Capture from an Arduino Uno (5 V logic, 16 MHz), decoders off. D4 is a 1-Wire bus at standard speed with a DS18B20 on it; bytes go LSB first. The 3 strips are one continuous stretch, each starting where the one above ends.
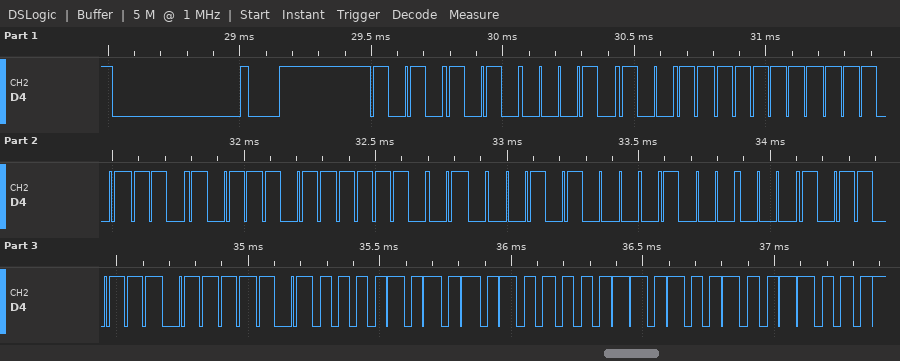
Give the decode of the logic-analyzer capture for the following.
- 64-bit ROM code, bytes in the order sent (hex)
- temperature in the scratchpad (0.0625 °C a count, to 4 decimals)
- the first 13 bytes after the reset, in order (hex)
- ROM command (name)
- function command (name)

28 FF 77 DD 4F 14 02 ED
85.0000 °C
55 28 FF 77 DD 4F 14 02 ED BE 50 05 4B
Match ROM
Read Scratchpad
